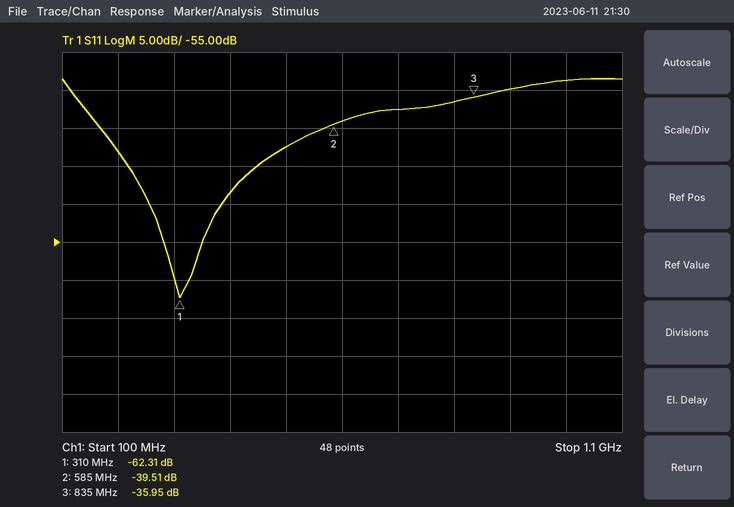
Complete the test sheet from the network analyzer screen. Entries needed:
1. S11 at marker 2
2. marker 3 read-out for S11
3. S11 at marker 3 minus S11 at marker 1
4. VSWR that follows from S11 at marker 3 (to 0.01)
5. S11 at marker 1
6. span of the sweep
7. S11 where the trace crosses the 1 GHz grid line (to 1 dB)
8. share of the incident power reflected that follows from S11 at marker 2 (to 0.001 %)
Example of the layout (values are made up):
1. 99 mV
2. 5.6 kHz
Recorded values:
1. -39.51 dB
2. -35.95 dB
3. 26.36 dB
4. 1.03
5. -62.31 dB
6. 1 GHz
7. -34 dB
8. 0.011 %
